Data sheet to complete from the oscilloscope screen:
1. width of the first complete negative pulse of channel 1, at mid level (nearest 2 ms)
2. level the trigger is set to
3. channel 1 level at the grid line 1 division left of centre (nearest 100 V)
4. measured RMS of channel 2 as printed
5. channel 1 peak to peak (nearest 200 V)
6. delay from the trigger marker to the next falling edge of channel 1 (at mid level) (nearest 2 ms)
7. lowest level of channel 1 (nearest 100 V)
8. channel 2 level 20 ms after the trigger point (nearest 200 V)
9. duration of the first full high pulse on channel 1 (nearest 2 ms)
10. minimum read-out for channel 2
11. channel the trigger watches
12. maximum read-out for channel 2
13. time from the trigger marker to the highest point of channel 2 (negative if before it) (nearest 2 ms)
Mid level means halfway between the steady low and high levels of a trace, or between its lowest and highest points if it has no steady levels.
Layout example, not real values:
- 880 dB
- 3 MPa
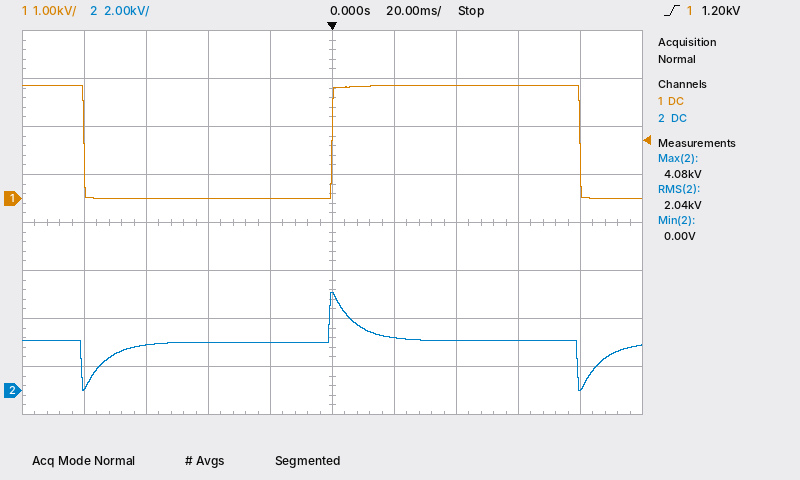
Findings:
- 80 ms
- 1.20 kV
- 0.0 kV
- 2.04 kV
- 2.4 kV
- 80 ms
- 0.0 kV
- 2.2 kV
- 80 ms
- 0.00 V
- channel 1
- 4.08 kV
- 0 ms
